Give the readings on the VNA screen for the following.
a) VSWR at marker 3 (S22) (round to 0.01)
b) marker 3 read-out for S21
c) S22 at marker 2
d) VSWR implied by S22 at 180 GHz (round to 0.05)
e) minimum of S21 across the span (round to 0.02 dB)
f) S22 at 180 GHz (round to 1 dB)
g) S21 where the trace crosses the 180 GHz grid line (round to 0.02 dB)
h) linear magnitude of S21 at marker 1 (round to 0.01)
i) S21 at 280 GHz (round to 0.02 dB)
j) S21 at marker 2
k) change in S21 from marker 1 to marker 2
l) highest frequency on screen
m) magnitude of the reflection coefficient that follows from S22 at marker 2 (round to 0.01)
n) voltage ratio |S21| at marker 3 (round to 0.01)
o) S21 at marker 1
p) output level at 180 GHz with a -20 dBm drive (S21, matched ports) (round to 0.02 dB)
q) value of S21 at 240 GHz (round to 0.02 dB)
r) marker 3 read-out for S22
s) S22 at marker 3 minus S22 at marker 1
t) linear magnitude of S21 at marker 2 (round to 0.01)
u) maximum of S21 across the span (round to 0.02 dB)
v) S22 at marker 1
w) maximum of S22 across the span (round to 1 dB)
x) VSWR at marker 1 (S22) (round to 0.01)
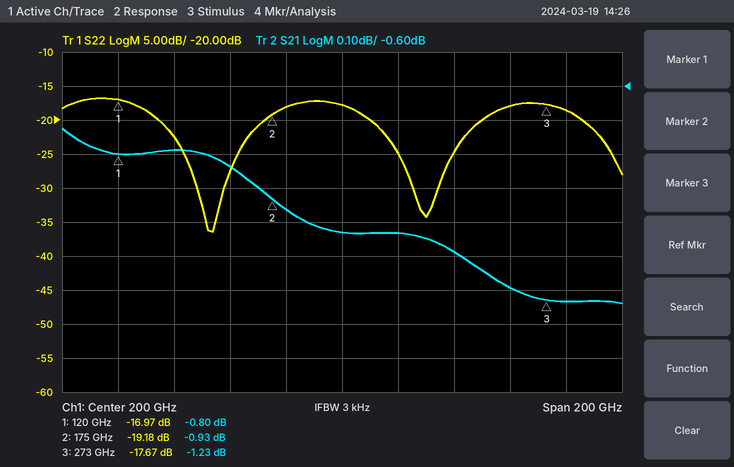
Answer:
1.30
-1.23 dB
-19.18 dB
1.30
-1.24 dB
-18 dB
-0.96 dB
0.91
-1.24 dB
-0.93 dB
-0.13 dB
300 GHz
0.11
0.87
-0.80 dB
-20.96 dBm
-1.08 dB
-17.67 dB
-0.70 dB
0.90
-0.72 dB
-16.97 dB
-17 dB
1.33
